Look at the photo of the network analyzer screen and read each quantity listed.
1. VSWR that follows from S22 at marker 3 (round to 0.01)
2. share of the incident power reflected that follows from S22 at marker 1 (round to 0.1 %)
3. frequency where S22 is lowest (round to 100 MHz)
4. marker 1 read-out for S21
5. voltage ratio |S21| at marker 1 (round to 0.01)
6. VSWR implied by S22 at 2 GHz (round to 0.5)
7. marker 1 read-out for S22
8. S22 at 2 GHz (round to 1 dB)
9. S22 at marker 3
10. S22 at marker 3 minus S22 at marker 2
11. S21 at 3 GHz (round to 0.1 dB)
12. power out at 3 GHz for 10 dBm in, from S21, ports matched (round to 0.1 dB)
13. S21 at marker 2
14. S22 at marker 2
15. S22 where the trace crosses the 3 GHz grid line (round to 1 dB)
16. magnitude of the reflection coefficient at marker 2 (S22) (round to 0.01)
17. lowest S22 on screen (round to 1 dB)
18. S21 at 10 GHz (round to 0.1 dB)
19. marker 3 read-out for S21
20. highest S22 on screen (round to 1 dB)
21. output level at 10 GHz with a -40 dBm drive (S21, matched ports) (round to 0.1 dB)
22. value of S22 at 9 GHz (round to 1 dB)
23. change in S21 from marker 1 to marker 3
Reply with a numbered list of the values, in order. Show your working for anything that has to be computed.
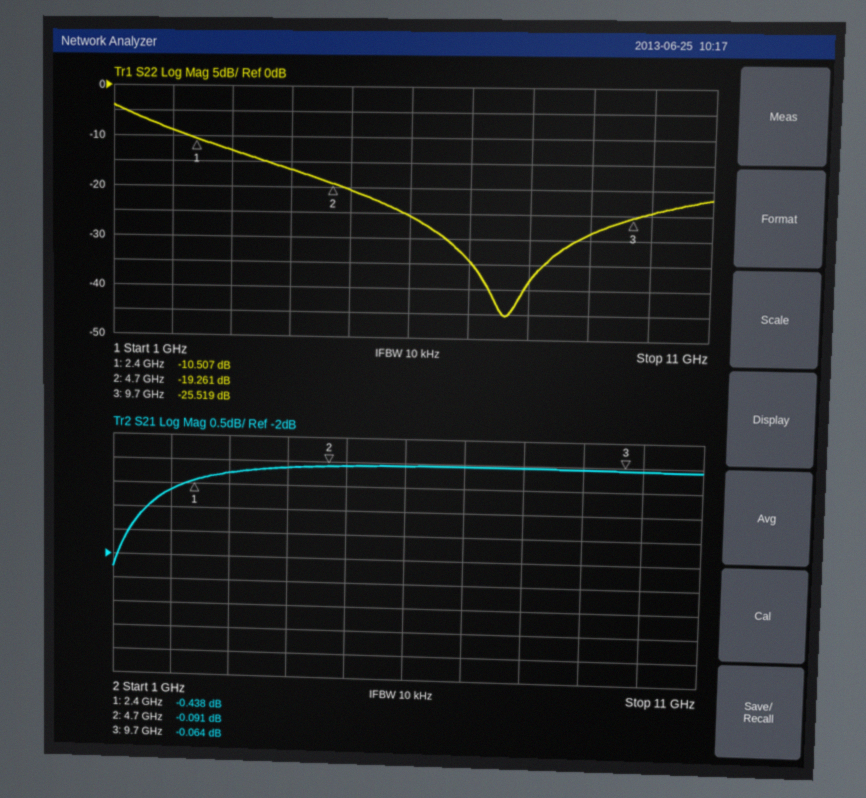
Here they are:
1. (1 + 0.0530)/(1 − 0.0530) ≈ 1.11
2. 10^(-10.507/10) ≈ 8.9 %
3. 7.6 GHz
4. -0.438 dB
5. 10^(-0.438/20) ≈ 0.95
6. |Γ| = 10^(-9/20) = 0.3548; VSWR = (1 + 0.3548)/(1 − 0.3548) ≈ 2.10, so 2.0 to the nearest 0.5
7. -10.507 dB
8. -9 dB
9. -25.519 dB
10. -25.519 − (-19.261) = -6.258 dB
11. -0.3 dB
12. 10 dBm + (-0.3 dB) = 9.7 dBm
13. -0.091 dB
14. -19.261 dB
15. -13 dB
16. 10^(-19.261/20) ≈ 0.11
17. -45 dB
18. -0.1 dB
19. -0.064 dB
20. -4 dB
21. -40 dBm + (-0.1 dB) = -40.1 dBm
22. -29 dB
23. -0.064 − (-0.438) = 0.374 dB
